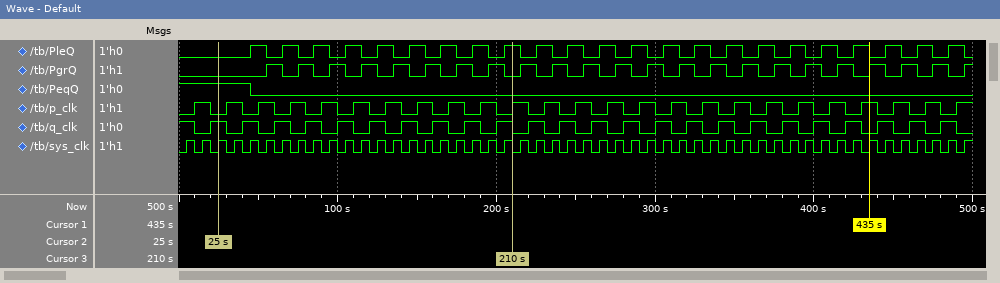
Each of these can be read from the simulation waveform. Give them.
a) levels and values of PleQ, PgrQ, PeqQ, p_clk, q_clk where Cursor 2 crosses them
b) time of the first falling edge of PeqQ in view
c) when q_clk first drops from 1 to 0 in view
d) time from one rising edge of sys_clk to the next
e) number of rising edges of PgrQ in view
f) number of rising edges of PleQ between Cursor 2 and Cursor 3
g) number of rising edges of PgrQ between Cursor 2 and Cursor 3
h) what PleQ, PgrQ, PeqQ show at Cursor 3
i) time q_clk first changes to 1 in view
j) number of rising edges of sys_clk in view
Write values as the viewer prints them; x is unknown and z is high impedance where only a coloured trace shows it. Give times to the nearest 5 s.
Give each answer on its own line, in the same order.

PleQ=0, PgrQ=0, PeqQ=1, p_clk=0, q_clk=1
45 s
10 s
10 s
23
9
8
PleQ=1, PgrQ=0, PeqQ=0
20 s
50
